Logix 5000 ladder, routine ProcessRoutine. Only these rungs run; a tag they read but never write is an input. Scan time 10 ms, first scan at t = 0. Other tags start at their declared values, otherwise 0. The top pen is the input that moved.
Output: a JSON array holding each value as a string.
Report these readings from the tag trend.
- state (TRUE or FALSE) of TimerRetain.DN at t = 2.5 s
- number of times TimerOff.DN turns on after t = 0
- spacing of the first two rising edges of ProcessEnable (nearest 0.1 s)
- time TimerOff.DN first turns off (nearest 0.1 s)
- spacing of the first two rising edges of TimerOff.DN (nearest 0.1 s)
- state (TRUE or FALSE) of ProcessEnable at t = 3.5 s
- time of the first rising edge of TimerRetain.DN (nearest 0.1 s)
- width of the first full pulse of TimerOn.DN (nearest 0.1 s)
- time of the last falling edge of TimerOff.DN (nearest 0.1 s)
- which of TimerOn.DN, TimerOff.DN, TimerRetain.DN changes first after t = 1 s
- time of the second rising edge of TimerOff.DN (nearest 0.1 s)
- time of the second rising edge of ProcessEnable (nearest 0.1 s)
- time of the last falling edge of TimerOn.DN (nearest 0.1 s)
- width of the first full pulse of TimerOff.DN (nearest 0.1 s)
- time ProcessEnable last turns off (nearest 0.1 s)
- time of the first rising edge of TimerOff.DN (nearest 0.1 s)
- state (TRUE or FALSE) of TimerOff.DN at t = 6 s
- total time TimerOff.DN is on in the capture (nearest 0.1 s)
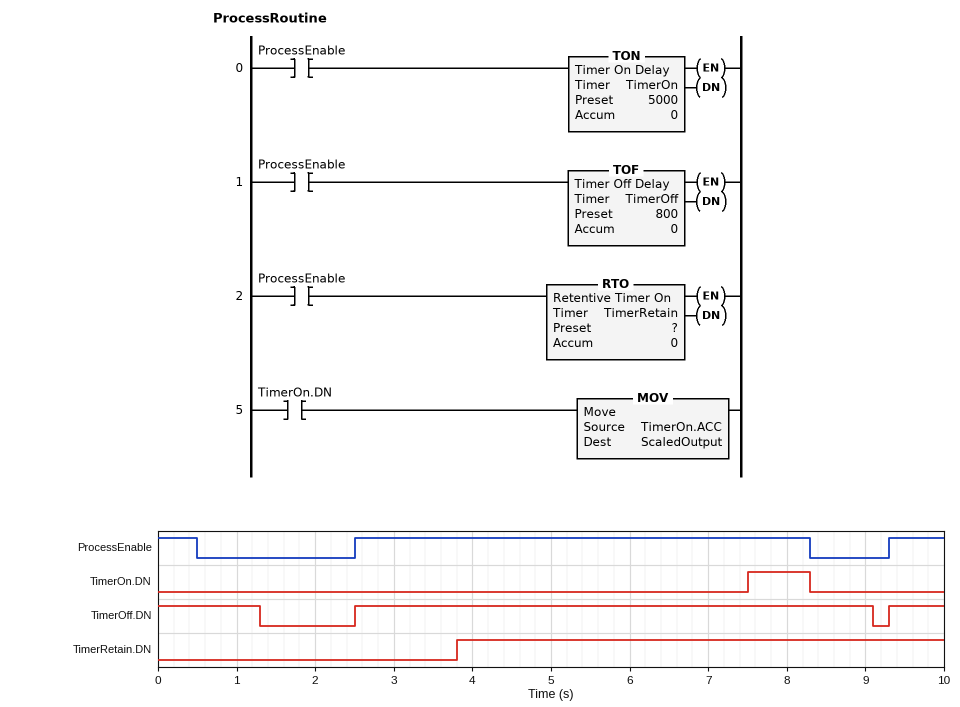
["FALSE", "2", "6.8 s", "1.3 s", "6.8 s", "TRUE", "3.8 s", "0.8 s", "9.1 s", "TimerOff.DN", "9.3 s", "9.3 s", "8.3 s", "6.6 s", "8.3 s", "2.5 s", "TRUE", "8.6 s"]
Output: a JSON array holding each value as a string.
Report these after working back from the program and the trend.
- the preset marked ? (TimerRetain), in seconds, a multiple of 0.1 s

["1.8 s"]
